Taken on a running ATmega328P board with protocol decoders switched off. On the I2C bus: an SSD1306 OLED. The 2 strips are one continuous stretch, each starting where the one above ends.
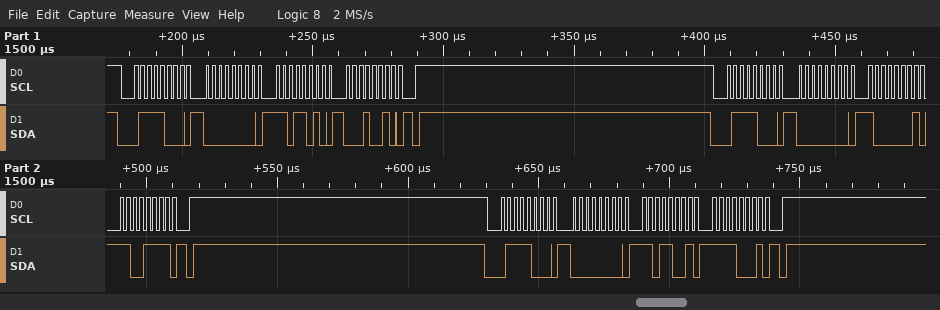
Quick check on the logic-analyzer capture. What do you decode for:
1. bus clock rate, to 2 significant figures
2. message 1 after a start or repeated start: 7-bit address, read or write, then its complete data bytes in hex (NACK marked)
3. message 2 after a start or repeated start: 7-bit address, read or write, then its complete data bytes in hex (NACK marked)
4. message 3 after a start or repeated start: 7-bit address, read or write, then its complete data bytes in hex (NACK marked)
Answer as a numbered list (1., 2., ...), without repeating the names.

1. 400 kHz
2. 0x3C write: 00 DA 12
3. 0x3C write: 00 81 CF
4. 0x3C write: 00 D9 F1
